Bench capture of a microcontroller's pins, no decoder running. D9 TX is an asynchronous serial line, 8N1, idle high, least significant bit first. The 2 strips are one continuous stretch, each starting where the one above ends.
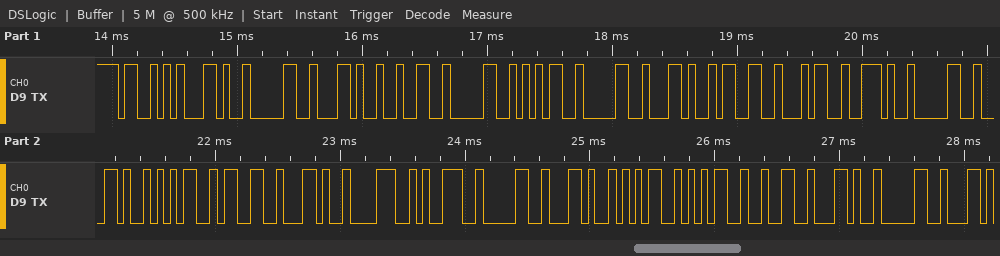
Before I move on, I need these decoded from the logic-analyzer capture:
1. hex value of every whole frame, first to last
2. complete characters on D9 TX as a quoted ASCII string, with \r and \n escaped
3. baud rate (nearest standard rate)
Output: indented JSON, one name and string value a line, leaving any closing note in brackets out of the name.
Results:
{
  "hex value of every whole frame, first to last": "0x53 0x2C 0x30 0x2C 0x32 0x30 0x35 0x30 0x2C 0x33 0x34 0x2E 0x30 0x2C 0x35 0x33 0x2C 0x38 0x39 0x30 0x2C 0x35 0x35 0x32 0x2C 0x30",
  "complete characters on D9 TX as a quoted ASCII string, with \\r and \\n escaped": "\"S,0,2050,34.0,53,890,552,0\"",
  "baud rate": "19200 baud"
}
